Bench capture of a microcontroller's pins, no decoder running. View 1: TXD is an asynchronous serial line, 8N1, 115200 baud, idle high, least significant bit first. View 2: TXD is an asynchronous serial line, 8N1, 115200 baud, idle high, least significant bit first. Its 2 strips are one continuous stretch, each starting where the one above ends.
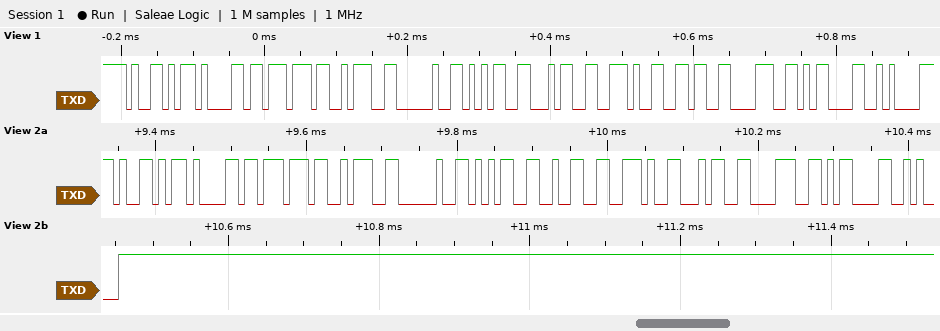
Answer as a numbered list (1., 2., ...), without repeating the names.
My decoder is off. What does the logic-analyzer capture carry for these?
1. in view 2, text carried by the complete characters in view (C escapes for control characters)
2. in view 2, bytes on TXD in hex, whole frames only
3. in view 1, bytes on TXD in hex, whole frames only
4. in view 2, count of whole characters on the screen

1. "Yaw: 52.48\r\n"
2. 59 61 77 3A 20 35 32 2E 34 38 0D 0A
3. 59 61 77 3A 20 35 34 2E 36 38 0D 0A
4. 12
